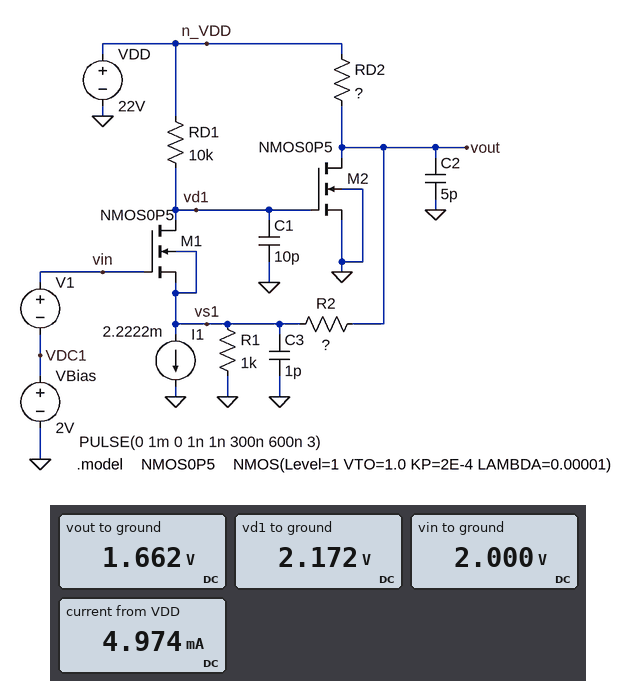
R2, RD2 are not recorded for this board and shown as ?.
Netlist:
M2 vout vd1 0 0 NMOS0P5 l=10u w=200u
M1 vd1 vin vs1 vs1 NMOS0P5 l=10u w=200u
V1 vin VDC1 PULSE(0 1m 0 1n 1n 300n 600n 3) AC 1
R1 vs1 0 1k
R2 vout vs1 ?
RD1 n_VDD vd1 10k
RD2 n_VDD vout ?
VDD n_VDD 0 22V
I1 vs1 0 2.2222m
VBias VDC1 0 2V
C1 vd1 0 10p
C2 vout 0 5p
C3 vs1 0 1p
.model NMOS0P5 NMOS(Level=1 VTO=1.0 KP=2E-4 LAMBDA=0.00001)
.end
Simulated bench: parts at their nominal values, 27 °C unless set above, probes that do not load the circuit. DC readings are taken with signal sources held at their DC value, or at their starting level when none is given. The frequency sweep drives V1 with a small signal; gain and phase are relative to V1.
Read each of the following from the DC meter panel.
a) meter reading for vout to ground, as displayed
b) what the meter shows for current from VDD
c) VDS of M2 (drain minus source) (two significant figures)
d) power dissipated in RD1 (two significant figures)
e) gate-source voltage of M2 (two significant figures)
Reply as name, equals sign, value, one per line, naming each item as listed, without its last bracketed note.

meter reading for vout to ground, as displayed = 1.662 V
what the meter shows for current from VDD = 4.974 mA
VDS of M2 (drain minus source) = 1.7 V
power dissipated in RD1 = 39 mW
gate-source voltage of M2 = 2.2 V
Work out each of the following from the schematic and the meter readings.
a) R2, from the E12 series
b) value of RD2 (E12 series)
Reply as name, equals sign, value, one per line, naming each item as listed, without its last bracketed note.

R2, from the E12 series = 6.8 kΩ
value of RD2 = 6.8 kΩ
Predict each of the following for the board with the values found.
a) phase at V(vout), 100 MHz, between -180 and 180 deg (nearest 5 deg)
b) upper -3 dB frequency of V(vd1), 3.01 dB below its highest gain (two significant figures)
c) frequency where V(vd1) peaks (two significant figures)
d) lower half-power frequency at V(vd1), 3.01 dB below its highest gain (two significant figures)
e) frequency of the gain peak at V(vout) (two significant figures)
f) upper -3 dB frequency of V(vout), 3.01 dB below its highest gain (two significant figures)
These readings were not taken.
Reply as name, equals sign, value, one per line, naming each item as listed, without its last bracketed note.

phase at V(vout), 100 MHz, between -180 and 180 deg = -145 deg
upper -3 dB frequency of V(vd1), 3.01 dB below its highest gain = 22 MHz
frequency where V(vd1) peaks = 17 MHz
lower half-power frequency at V(vd1), 3.01 dB below its highest gain = 12 MHz
frequency of the gain peak at V(vout) = 15 MHz
upper -3 dB frequency of V(vout), 3.01 dB below its highest gain = 20 MHz
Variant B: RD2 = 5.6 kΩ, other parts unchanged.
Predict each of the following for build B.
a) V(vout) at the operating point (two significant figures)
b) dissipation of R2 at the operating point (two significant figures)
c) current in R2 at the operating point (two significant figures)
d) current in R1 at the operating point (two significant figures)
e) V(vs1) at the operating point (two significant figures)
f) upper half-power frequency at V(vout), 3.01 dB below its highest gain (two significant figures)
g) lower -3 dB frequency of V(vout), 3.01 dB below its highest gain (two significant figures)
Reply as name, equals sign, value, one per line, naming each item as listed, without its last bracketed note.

V(vout) at the operating point = 1.8 V
dissipation of R2 at the operating point = 460 µW
current in R2 at the operating point = 260 µA
current in R1 at the operating point = 7.4 µA
V(vs1) at the operating point = 7.4 mV
upper half-power frequency at V(vout), 3.01 dB below its highest gain = 21 MHz
lower -3 dB frequency of V(vout), 3.01 dB below its highest gain = 7.7 MHz
